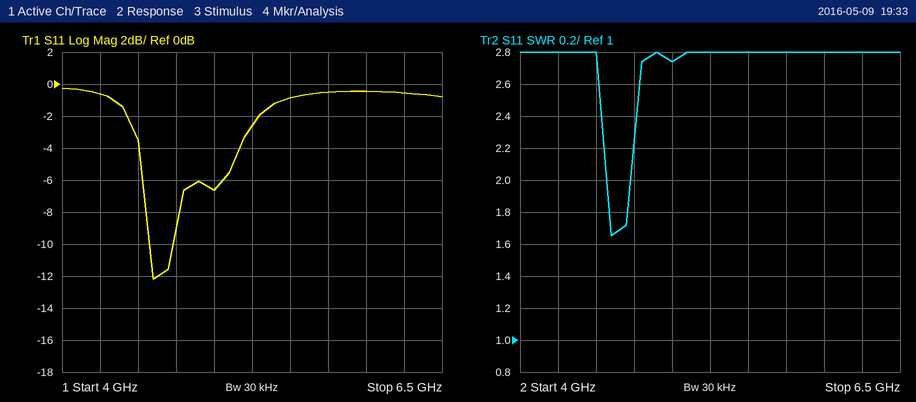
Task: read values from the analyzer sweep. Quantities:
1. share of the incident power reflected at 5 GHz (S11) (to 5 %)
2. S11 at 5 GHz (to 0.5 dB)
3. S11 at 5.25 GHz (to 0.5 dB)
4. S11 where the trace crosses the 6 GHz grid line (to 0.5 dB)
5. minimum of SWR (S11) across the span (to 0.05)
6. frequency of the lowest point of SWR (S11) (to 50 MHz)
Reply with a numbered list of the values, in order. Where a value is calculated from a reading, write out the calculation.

1. 10^(-6.5/10) ≈ 22.4 %, so 20 % to the nearest 5 %
2. -6.5 dB
3. -2.5 dB
4. -0.5 dB
5. 1.65
6. 4.60 GHz
